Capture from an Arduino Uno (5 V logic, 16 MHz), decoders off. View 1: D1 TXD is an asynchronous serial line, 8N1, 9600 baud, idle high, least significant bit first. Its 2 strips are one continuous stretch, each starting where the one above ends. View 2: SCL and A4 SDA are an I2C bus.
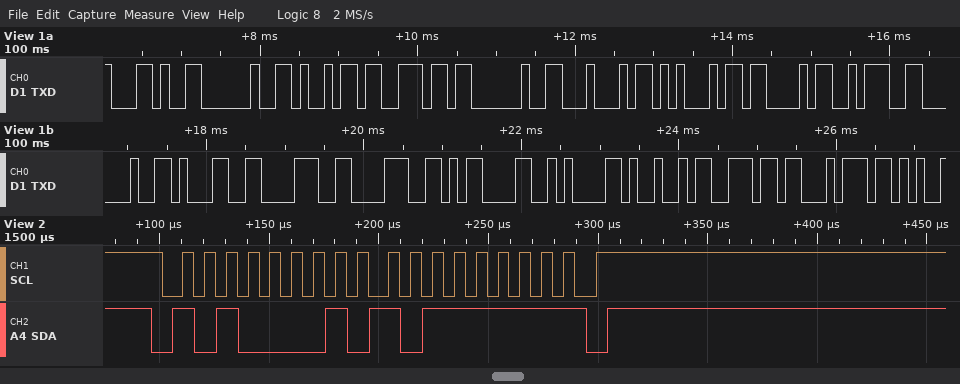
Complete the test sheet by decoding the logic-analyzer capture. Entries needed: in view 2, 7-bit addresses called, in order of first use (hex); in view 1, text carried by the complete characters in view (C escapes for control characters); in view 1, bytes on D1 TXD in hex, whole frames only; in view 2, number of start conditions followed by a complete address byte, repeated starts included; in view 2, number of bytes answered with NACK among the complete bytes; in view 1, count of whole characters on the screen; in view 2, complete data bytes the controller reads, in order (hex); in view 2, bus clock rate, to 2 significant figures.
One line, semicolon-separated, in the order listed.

0x50; ", in DEC: 188\r\nInt"; 2C 20 69 6E 20 44 45 43 3A 20 31 38 38 0D 0A 49 6E 74; 1; 1; 18; BF; 100 kHz
